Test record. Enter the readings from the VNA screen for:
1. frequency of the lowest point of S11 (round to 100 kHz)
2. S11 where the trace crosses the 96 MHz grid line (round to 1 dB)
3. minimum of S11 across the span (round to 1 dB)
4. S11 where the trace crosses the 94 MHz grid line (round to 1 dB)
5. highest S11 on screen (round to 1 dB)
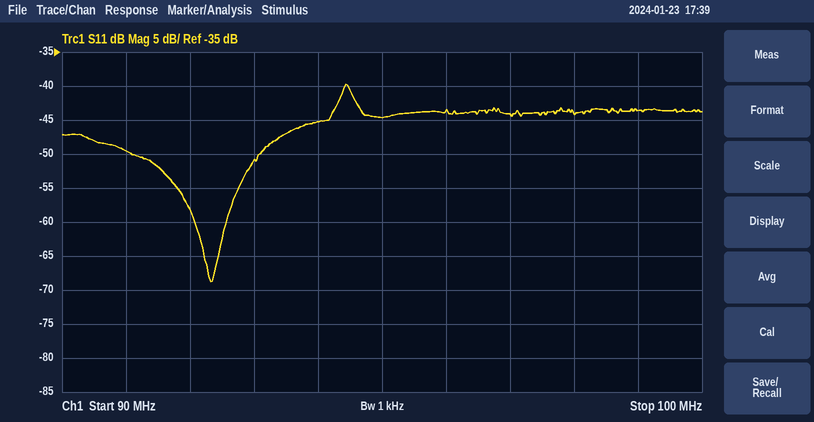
92.3 MHz
-44 dB
-69 dB
-45 dB
-40 dB
